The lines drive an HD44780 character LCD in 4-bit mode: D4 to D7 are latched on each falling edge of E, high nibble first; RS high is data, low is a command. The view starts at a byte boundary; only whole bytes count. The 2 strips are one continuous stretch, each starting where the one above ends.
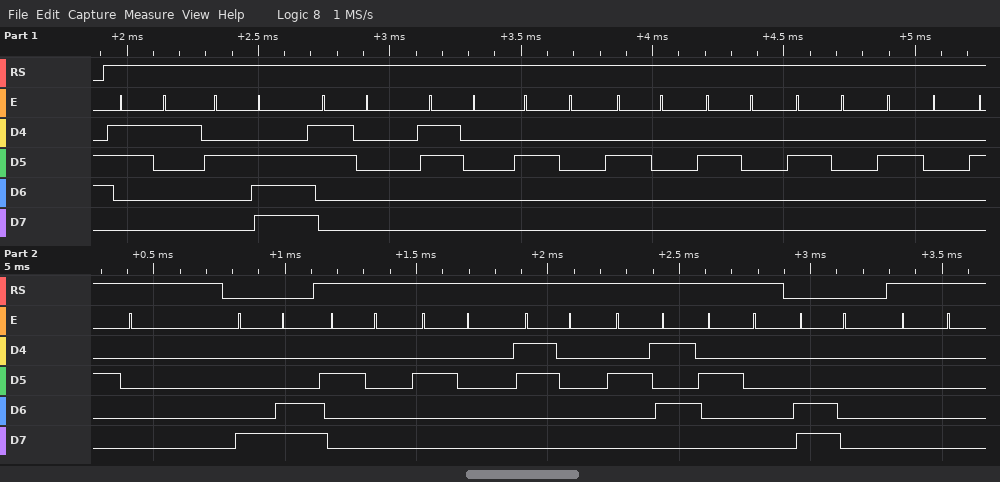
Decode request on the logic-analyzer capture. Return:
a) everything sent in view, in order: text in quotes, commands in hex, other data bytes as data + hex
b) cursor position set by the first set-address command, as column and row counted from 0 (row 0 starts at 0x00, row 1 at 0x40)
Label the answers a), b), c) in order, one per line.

a) "1.00      " 0x8C "  0% " 0xC0 data 00
b) column 12, row 0
